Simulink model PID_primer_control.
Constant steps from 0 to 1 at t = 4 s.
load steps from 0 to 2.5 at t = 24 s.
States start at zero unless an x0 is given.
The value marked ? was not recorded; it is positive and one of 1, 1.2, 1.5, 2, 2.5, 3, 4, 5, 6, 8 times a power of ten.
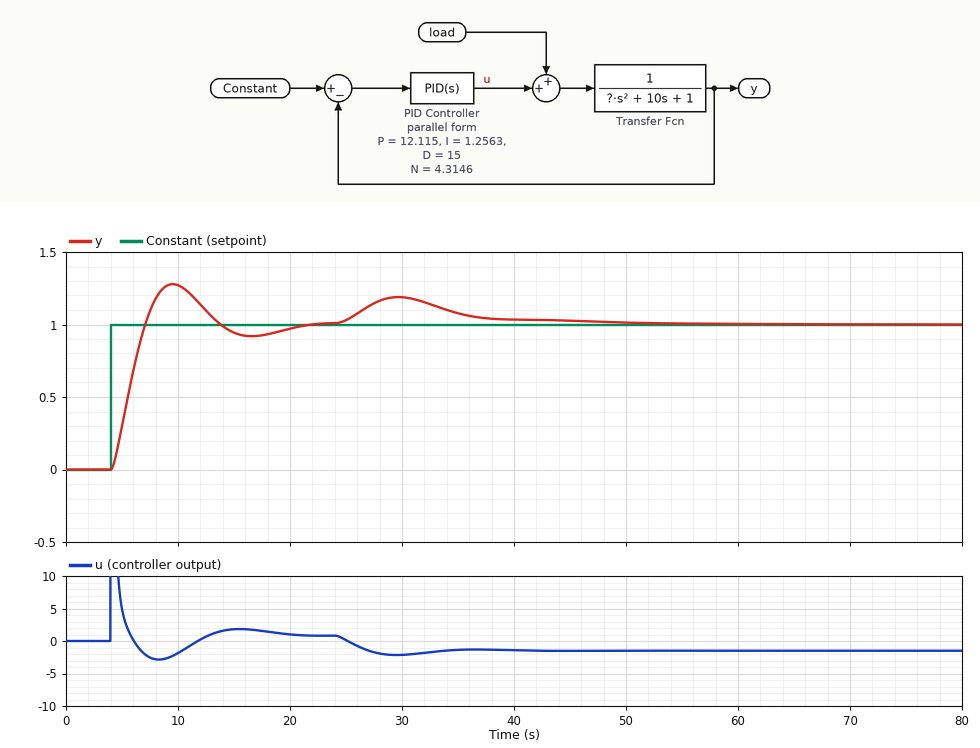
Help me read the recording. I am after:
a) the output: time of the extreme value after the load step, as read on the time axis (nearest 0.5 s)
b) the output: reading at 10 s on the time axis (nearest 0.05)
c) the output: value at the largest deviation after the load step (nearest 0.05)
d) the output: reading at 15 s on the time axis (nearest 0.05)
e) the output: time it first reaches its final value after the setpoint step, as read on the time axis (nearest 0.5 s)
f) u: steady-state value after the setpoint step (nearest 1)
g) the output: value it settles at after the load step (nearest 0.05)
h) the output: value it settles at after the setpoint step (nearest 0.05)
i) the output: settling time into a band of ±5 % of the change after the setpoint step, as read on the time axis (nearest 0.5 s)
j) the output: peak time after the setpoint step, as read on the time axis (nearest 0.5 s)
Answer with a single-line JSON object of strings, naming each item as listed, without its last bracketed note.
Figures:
{"the output: time of the extreme value after the load step, as read on the time axis": "29.5 s", "the output: reading at 10 s on the time axis": "1.25", "the output: value at the largest deviation after the load step": "1.20", "the output: reading at 15 s on the time axis": "0.95", "the output: time it first reaches its final value after the setpoint step, as read on the time axis": "7.0 s", "u: steady-state value after the setpoint step": "1", "the output: value it settles at after the load step": "1.00", "the output: value it settles at after the setpoint step": "1.00", "the output: settling time into a band of ±5 % of the change after the setpoint step, as read on the time axis": "19.0 s", "the output: peak time after the setpoint step, as read on the time axis": "9.5 s"}
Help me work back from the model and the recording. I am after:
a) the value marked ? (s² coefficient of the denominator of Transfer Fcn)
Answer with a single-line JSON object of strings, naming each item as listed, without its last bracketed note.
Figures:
{"the value marked ?": "50"}
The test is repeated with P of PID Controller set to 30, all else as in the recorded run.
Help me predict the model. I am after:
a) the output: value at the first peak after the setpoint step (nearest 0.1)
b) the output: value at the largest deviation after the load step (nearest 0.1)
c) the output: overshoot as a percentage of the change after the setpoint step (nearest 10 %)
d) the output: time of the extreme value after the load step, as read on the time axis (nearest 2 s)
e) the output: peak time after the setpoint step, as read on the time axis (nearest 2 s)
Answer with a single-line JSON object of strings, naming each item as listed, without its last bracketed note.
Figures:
{"the output: value at the first peak after the setpoint step": "1.4", "the output: value at the largest deviation after the load step": "1.1", "the output: overshoot as a percentage of the change after the setpoint step": "40 %", "the output: time of the extreme value after the load step, as read on the time axis": "28 s", "the output: peak time after the setpoint step, as read on the time axis": "8 s"}
